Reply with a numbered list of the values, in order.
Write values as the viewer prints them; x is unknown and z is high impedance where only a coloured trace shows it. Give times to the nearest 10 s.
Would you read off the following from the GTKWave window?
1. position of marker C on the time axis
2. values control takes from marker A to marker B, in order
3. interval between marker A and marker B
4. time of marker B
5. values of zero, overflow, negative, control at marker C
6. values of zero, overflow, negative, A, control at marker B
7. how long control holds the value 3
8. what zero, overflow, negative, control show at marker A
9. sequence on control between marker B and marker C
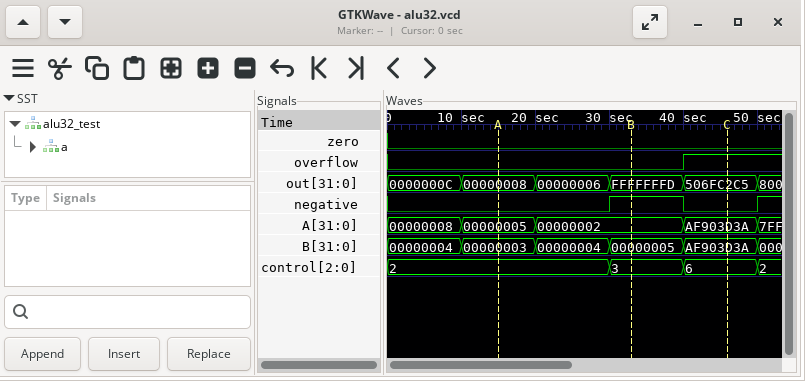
1. 50 s
2. 2, 3
3. 20 s
4. 30 s
5. zero=0, overflow=1, negative=0, control=6
6. zero=0, overflow=0, negative=1, A=00000002, control=3
7. 10 s
8. zero=0, overflow=0, negative=0, control=2
9. 3, 6
